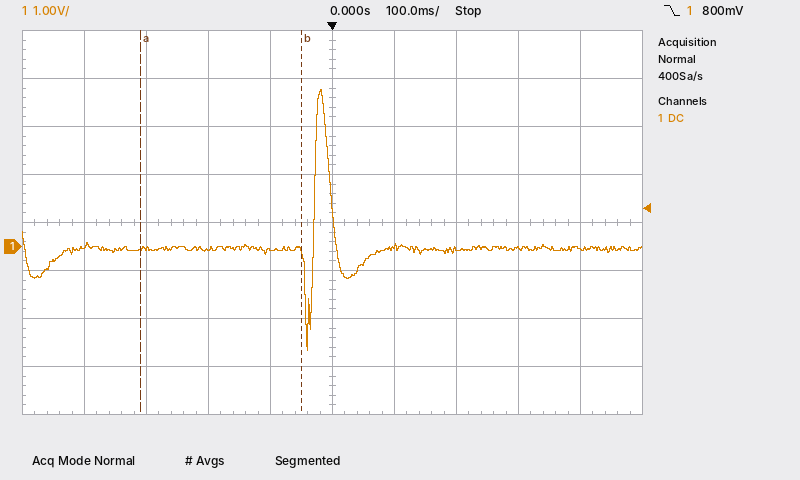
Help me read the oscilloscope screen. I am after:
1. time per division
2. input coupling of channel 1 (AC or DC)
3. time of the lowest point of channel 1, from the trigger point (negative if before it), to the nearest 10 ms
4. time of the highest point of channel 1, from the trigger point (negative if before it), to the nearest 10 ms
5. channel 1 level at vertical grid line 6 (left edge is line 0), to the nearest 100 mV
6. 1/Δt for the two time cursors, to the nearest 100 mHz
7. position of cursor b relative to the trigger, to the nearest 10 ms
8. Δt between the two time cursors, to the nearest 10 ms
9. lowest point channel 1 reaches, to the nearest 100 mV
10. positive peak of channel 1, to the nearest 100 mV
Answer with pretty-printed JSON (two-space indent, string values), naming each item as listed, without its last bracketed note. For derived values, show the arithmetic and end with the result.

{
  "time per division": "100 ms",
  "input coupling of channel 1": "DC",
  "time of the lowest point of channel 1, from the trigger point (negative if before it), to the nearest 10 ms": "-40 ms",
  "time of the highest point of channel 1, from the trigger point (negative if before it), to the nearest 10 ms": "-20 ms",
  "channel 1 level at vertical grid line 6 (left edge is line 0), to the nearest 100 mV": "0.0 V",
  "1/Δt for the two time cursors, to the nearest 100 mHz": "1 / 260 ms ≈ 3.8 Hz",
  "position of cursor b relative to the trigger, to the nearest 10 ms": "-50 ms",
  "Δt between the two time cursors, to the nearest 10 ms": "260 ms",
  "lowest point channel 1 reaches, to the nearest 100 mV": "-2.2 V",
  "positive peak of channel 1, to the nearest 100 mV": "3.3 V"
}
